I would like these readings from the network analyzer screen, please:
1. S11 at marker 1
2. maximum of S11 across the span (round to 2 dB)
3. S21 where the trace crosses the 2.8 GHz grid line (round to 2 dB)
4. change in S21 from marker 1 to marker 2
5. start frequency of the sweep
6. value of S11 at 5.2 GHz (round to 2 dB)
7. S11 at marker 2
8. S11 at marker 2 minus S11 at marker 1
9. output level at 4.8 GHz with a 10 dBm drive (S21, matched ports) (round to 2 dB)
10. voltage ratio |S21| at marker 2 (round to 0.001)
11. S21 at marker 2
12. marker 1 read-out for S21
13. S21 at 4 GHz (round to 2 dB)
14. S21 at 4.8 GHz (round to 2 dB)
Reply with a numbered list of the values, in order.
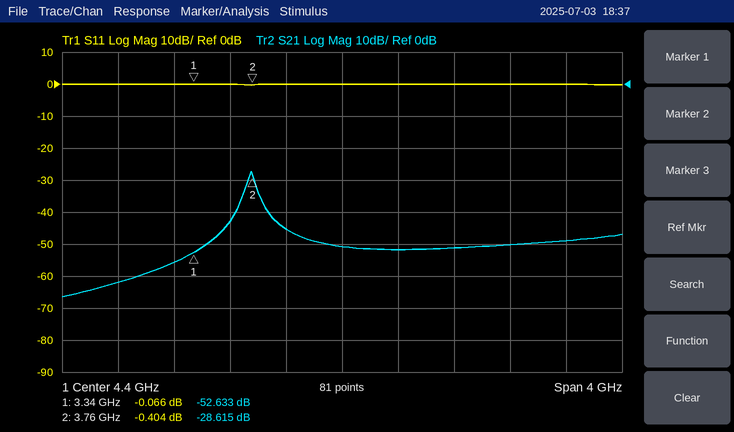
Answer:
1. -0.066 dB
2. 0 dB
3. -62 dB
4. 24.018 dB
5. 2.4 GHz
6. 0 dB
7. -0.404 dB
8. -0.338 dB
9. -42 dBm
10. 0.037
11. -28.615 dB
12. -52.633 dB
13. -46 dB
14. -52 dB
